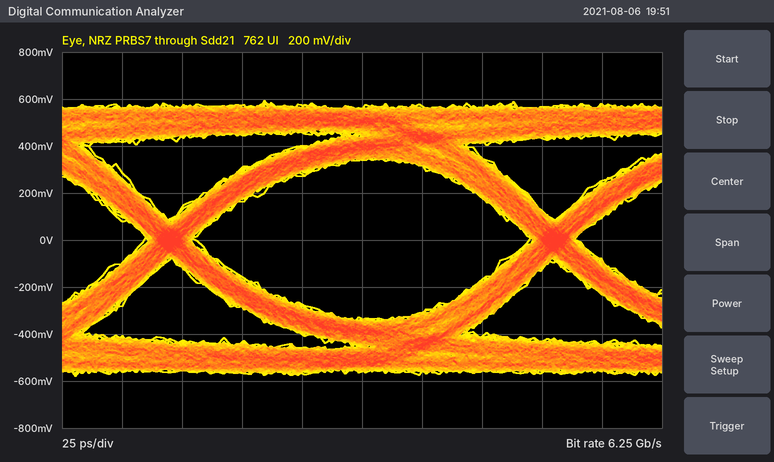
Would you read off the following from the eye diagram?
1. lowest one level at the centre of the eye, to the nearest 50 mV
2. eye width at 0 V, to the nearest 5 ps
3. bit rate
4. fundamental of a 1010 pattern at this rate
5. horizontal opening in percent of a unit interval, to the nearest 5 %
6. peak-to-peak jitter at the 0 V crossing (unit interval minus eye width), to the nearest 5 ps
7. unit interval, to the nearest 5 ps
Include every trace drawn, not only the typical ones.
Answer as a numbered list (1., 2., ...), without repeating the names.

1. 350 mV
2. 140 ps
3. 6.25 Gb/s
4. 3.125 GHz
5. 85 %
6. 20 ps
7. 160 ps
